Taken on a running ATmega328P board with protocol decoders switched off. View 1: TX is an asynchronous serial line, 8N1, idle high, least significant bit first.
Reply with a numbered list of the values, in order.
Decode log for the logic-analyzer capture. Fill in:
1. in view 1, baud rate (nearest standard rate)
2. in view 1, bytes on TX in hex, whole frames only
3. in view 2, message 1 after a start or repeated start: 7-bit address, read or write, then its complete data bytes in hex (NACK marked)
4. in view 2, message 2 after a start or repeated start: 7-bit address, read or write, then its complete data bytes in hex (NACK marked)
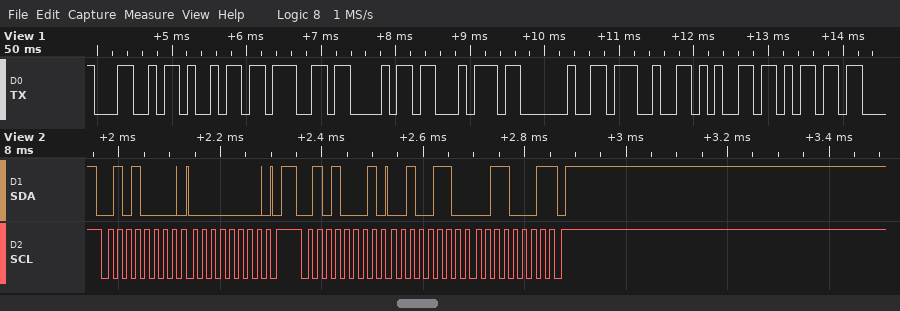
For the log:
1. 9600 baud
2. 4C 69 67 68 74 20 27 65 6D
3. 0x28 write: 00
4. 0x28 read: 26 31 NACK
